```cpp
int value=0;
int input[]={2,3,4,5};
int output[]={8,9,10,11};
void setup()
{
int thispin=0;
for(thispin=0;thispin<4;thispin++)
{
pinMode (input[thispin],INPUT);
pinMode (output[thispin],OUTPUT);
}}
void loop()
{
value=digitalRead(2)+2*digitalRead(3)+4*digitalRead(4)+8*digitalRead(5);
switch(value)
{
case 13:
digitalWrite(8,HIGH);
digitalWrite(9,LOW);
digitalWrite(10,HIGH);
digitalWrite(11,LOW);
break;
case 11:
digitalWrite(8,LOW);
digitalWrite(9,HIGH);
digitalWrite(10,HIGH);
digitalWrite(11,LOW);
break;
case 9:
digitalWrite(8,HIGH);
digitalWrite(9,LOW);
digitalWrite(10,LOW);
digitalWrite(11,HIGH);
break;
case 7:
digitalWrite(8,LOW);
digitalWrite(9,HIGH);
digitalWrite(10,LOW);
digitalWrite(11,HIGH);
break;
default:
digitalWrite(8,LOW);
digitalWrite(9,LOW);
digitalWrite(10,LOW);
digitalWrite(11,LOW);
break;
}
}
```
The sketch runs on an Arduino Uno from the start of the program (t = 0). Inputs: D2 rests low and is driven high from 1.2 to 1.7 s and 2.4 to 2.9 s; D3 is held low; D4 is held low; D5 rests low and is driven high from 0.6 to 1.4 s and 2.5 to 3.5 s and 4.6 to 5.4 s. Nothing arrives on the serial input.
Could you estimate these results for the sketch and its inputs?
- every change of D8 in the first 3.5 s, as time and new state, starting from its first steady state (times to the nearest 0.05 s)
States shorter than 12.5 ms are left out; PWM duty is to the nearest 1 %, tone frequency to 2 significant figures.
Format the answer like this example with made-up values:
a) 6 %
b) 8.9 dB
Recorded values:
a) 0 s low; 1.2 s high; 1.4 s low; 2.5 s high; 2.9 s low
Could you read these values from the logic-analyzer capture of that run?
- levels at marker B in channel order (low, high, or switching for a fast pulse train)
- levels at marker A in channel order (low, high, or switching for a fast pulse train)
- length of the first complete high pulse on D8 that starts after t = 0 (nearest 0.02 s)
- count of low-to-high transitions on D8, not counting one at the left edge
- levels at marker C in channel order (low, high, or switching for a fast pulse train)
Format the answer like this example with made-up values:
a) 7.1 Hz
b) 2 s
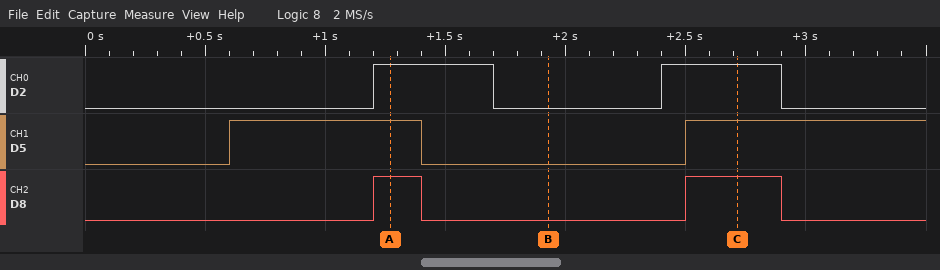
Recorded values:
a) D2 low, D5 low, D8 low
b) D2 high, D5 high, D8 high
c) 0.20 s
d) 2
e) D2 high, D5 high, D8 high
